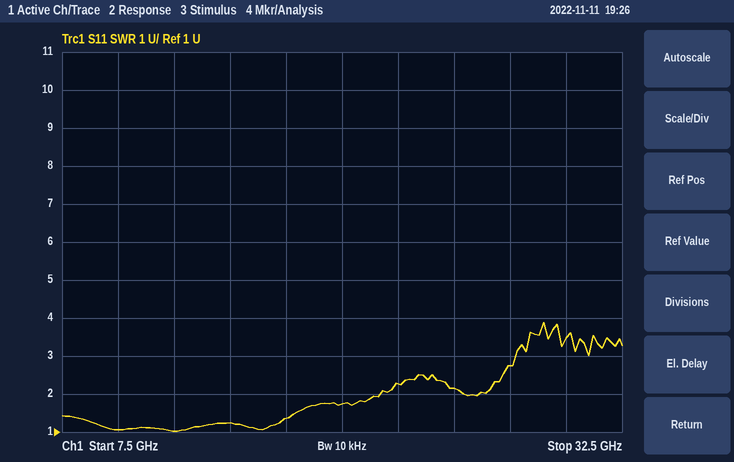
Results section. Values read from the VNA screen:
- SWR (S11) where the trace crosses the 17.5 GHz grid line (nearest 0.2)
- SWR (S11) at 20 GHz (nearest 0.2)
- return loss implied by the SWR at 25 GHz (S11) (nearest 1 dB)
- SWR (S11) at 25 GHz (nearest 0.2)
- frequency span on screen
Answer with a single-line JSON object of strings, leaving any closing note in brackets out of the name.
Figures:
{"SWR (S11) where the trace crosses the 17.5 GHz grid line": "1.4", "SWR (S11) at 20 GHz": "1.8", "return loss implied by the SWR at 25 GHz (S11)": "9 dB", "SWR (S11) at 25 GHz": "2.2", "frequency span on screen": "25 GHz"}
